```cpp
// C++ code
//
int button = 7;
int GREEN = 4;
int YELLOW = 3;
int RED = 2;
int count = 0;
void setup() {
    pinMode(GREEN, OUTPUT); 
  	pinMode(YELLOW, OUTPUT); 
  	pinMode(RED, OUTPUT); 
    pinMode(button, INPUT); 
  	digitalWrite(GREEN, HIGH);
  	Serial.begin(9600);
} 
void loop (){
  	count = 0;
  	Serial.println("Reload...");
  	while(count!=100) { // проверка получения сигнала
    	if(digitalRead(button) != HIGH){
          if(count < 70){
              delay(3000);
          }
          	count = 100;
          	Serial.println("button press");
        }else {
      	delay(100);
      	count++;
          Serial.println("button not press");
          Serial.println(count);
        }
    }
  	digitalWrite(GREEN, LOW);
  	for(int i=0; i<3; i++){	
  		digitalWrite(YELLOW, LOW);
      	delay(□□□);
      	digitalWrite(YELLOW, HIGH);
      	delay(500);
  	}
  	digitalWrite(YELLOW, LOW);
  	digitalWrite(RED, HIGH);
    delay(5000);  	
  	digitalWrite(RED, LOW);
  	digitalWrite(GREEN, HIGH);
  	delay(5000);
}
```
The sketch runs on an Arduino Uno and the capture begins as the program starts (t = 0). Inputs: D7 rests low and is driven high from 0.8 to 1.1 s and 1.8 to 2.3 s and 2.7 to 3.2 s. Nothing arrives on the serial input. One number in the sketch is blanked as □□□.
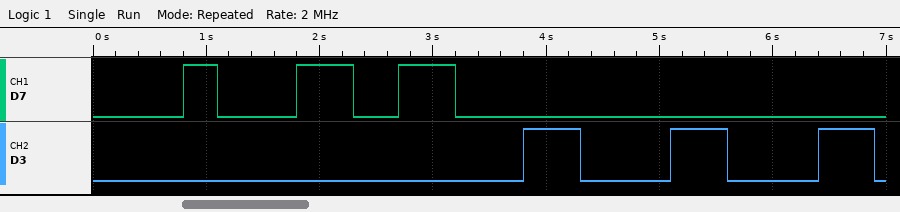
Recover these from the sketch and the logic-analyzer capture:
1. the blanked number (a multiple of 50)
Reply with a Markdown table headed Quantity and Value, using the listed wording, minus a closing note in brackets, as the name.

| Quantity | Value |
|---|---|
| the blanked number | 800 |
